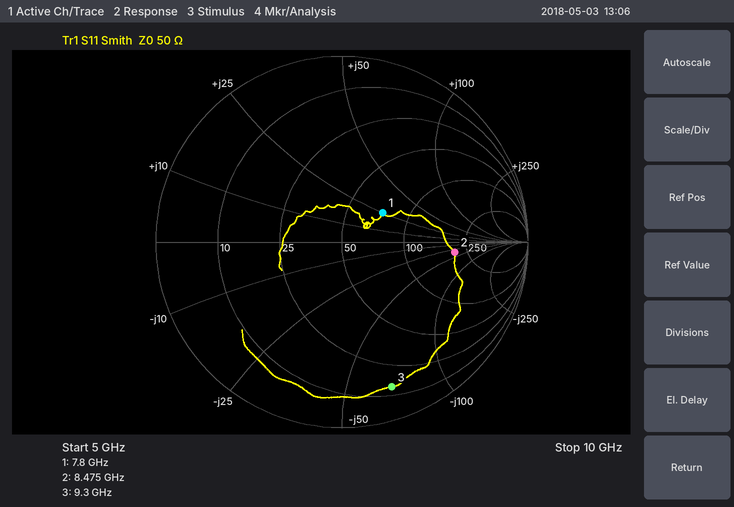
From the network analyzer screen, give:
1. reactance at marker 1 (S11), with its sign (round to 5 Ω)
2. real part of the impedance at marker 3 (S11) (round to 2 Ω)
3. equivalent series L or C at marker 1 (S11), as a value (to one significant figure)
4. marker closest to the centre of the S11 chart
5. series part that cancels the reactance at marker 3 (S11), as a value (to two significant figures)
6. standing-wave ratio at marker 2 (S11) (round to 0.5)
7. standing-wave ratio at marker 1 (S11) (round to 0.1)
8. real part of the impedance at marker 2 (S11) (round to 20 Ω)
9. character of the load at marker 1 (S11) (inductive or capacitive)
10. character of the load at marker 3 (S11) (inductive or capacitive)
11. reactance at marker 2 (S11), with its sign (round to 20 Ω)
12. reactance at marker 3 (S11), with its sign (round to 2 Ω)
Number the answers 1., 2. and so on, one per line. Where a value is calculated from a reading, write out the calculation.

1. +25 Ω
2. 14 Ω
3. L = 25 Ω/(2π × 7.8 GHz) ≈ 510 pH, so 500 pH to one significant figure
4. marker 1
5. L = 68 Ω/(2π × 9.3 GHz) ≈ 1.2 nH
6. 4.0
7. 1.7
8. 200 Ω
9. inductive
10. capacitive
11. -40 Ω
12. -68 Ω
